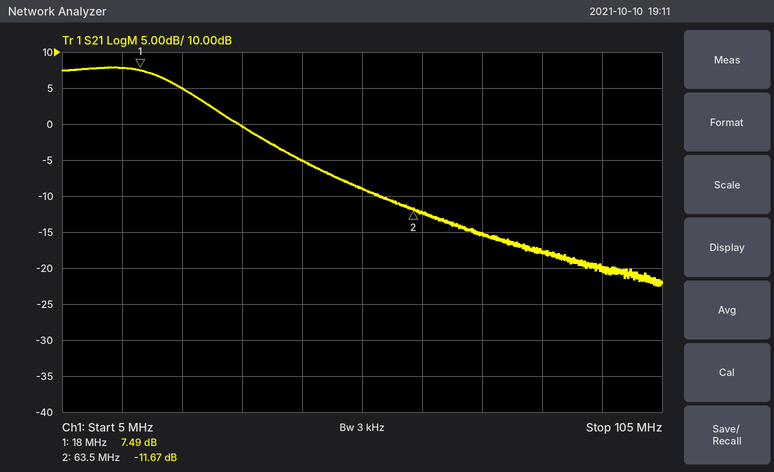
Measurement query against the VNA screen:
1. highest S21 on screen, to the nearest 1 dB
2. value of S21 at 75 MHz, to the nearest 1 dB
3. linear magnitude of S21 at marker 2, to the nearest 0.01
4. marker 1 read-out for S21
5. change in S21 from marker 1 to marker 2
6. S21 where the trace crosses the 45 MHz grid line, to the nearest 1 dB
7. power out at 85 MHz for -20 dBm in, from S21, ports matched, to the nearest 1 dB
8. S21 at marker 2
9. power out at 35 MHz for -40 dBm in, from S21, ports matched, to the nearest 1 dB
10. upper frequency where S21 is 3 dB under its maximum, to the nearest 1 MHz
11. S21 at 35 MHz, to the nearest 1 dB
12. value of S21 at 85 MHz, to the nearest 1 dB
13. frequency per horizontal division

8 dB
-15 dB
0.26
7.49 dB
-19.16 dB
-5 dB
-38 dBm
-11.67 dB
-40 dBm
25 MHz
0 dB
-18 dB
10 MHz
